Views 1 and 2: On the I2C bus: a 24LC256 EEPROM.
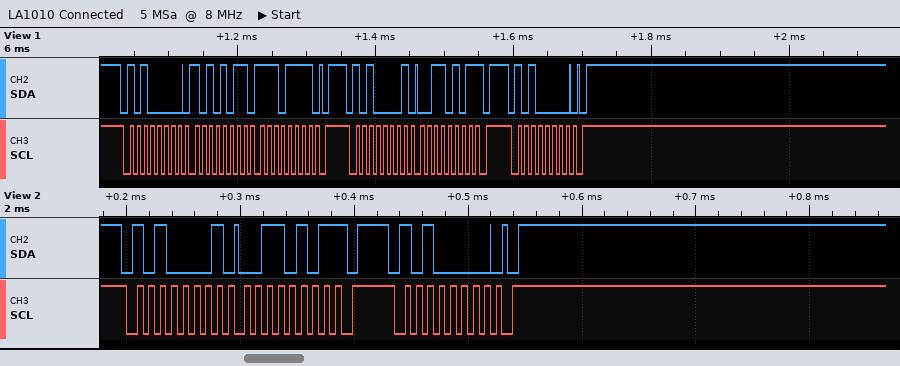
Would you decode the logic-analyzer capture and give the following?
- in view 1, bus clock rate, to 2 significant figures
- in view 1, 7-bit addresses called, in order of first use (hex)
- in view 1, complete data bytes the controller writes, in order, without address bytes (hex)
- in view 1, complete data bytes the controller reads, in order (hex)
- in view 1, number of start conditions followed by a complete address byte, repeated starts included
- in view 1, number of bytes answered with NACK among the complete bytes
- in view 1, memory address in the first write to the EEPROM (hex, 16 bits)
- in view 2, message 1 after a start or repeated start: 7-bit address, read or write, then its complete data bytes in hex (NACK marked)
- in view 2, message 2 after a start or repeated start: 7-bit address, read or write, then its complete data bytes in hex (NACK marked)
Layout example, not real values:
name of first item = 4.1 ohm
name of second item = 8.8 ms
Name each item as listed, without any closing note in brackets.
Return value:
in view 1, bus clock rate, to 2 significant figures = 100 kHz
in view 1, 7-bit addresses called, in order of first use = 0x50
in view 1, complete data bytes the controller writes, in order, without address bytes = AB EF
in view 1, complete data bytes the controller reads, in order = 35
in view 1, number of start conditions followed by a complete address byte, repeated starts included = 3
in view 1, number of bytes answered with NACK among the complete bytes = 1
in view 1, memory address in the first write to the EEPROM = 0xABEF
in view 2, message 1 after a start or repeated start: 7-bit address, read or write, then its complete data bytes in hex = 0x50 read: 35 NACK
in view 2, message 2 after a start or repeated start: 7-bit address, read or write, then its complete data bytes in hex = 0x50 write
